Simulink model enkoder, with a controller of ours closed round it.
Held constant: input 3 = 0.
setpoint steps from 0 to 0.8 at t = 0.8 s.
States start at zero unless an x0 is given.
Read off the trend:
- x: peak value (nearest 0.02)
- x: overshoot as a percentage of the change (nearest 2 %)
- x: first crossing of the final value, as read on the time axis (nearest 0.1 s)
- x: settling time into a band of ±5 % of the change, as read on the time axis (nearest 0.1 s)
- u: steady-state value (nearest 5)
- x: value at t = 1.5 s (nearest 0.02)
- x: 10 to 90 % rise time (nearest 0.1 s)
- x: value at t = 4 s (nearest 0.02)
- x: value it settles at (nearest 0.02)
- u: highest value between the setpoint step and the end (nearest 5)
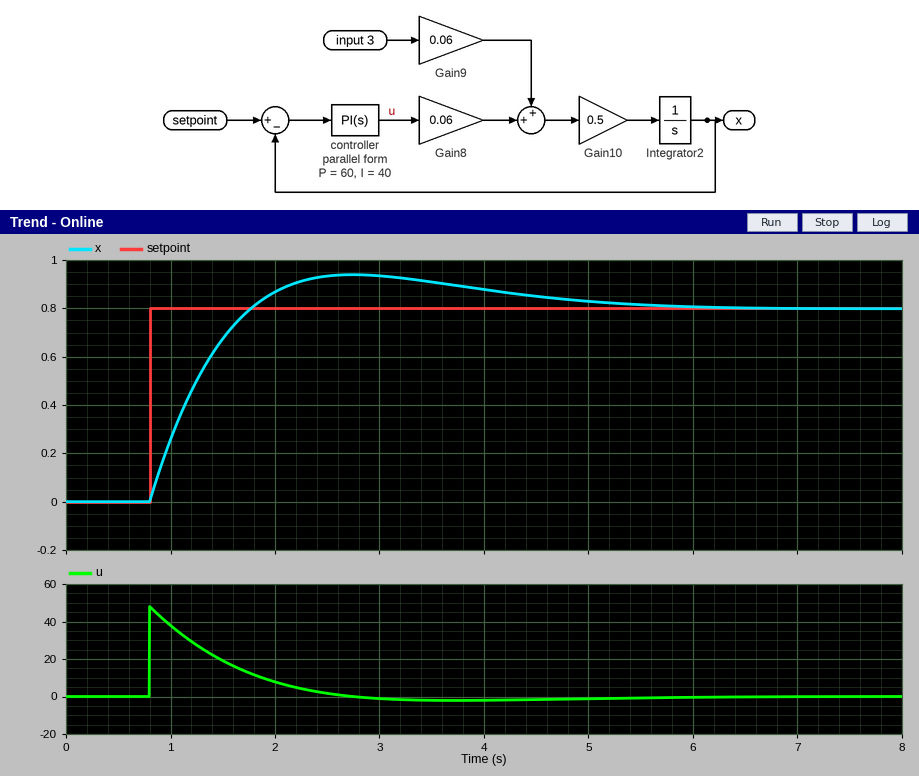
0.94
18 %
1.8 s
4.7 s
0
0.68
0.7 s
0.88
0.80
50
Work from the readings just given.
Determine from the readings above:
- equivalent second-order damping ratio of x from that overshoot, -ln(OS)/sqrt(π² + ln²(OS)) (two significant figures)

0.48
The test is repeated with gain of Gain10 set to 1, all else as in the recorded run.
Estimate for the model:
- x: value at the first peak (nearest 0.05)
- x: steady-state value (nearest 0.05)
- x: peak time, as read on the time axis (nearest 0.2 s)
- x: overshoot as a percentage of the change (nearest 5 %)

0.90
0.80
2.0 s
10 %
